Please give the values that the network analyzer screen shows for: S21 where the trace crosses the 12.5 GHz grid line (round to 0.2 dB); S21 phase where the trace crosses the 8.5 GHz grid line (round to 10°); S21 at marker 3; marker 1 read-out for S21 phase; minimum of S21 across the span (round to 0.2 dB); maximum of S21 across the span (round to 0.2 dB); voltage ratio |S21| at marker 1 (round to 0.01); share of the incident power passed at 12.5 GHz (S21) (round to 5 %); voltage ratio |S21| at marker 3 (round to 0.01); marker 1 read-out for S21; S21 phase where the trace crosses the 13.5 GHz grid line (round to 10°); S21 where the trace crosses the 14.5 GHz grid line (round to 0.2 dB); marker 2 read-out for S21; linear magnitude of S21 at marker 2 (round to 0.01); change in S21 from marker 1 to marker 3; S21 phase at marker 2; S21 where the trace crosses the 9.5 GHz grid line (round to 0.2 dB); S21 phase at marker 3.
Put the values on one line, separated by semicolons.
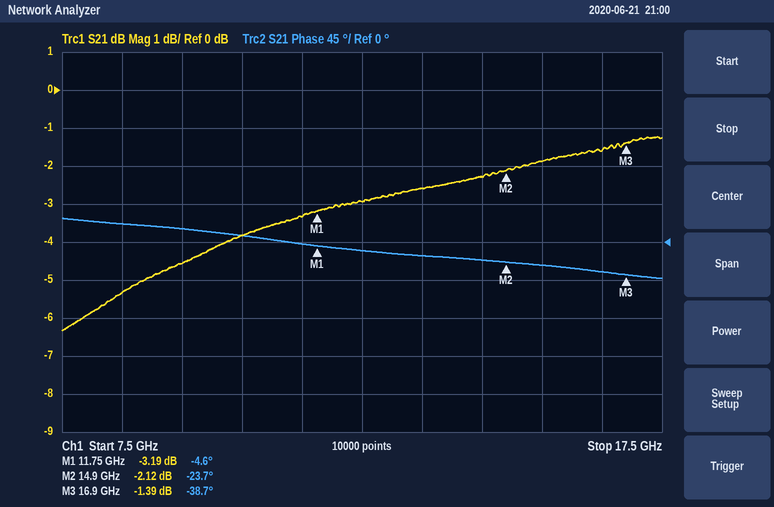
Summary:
-3.0 dB; 20°; -1.39 dB; -4.6°; -6.4 dB; -1.2 dB; 0.69; 50 %; 0.85; -3.19 dB; -20°; -2.2 dB; -2.12 dB; 0.78; 1.80 dB; -23.7°; -4.6 dB; -38.7°
